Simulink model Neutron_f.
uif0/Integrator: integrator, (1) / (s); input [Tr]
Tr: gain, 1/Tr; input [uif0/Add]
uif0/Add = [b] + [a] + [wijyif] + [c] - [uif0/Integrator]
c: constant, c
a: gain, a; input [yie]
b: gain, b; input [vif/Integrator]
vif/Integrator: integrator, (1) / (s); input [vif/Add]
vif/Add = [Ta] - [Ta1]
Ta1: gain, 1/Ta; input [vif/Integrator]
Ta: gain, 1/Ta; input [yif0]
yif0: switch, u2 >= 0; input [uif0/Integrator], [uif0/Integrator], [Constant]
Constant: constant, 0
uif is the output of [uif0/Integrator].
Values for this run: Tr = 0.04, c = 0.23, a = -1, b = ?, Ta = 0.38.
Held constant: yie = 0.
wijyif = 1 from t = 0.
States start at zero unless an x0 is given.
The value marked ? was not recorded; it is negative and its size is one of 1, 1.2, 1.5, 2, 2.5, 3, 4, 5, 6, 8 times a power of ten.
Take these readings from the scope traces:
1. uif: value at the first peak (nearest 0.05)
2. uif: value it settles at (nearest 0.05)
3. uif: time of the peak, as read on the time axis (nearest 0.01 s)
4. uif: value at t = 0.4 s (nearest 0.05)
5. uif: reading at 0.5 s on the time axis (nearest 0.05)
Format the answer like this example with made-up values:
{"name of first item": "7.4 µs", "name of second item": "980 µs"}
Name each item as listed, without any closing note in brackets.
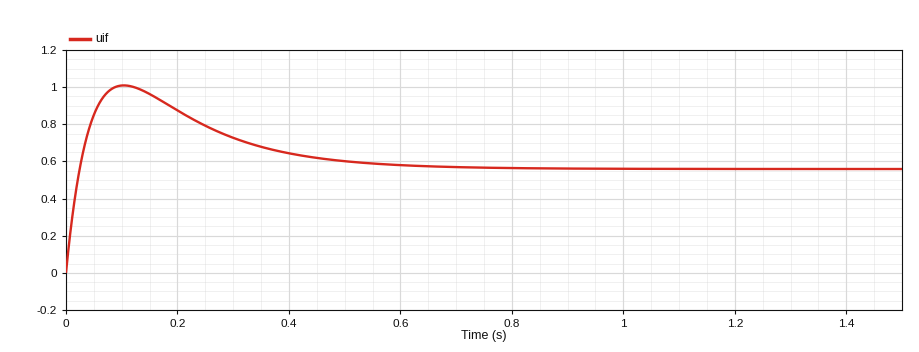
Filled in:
{"uif: value at the first peak": "1.00", "uif: value it settles at": "0.55", "uif: time of the peak, as read on the time axis": "0.10 s", "uif: value at t = 0.4 s": "0.65", "uif: reading at 0.5 s on the time axis": "0.60"}
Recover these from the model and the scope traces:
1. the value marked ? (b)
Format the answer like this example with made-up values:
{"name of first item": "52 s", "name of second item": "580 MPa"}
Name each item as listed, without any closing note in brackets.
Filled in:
{"the value marked ?": "-1.2"}
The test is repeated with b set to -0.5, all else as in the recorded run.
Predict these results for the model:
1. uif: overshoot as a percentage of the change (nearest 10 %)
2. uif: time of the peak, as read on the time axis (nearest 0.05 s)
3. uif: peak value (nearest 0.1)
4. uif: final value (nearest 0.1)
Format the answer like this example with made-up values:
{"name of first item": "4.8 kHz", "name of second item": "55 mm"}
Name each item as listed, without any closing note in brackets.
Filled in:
{"uif: overshoot as a percentage of the change": "30 %", "uif: time of the peak, as read on the time axis": "0.15 s", "uif: peak value": "1.1", "uif: final value": "0.8"}
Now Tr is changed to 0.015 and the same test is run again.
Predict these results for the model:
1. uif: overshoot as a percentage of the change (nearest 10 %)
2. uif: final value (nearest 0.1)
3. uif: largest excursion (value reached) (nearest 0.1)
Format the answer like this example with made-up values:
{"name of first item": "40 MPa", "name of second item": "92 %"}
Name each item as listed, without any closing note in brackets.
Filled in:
{"uif: overshoot as a percentage of the change": "100 %", "uif: final value": "0.6", "uif: largest excursion (value reached)": "1.1"}
